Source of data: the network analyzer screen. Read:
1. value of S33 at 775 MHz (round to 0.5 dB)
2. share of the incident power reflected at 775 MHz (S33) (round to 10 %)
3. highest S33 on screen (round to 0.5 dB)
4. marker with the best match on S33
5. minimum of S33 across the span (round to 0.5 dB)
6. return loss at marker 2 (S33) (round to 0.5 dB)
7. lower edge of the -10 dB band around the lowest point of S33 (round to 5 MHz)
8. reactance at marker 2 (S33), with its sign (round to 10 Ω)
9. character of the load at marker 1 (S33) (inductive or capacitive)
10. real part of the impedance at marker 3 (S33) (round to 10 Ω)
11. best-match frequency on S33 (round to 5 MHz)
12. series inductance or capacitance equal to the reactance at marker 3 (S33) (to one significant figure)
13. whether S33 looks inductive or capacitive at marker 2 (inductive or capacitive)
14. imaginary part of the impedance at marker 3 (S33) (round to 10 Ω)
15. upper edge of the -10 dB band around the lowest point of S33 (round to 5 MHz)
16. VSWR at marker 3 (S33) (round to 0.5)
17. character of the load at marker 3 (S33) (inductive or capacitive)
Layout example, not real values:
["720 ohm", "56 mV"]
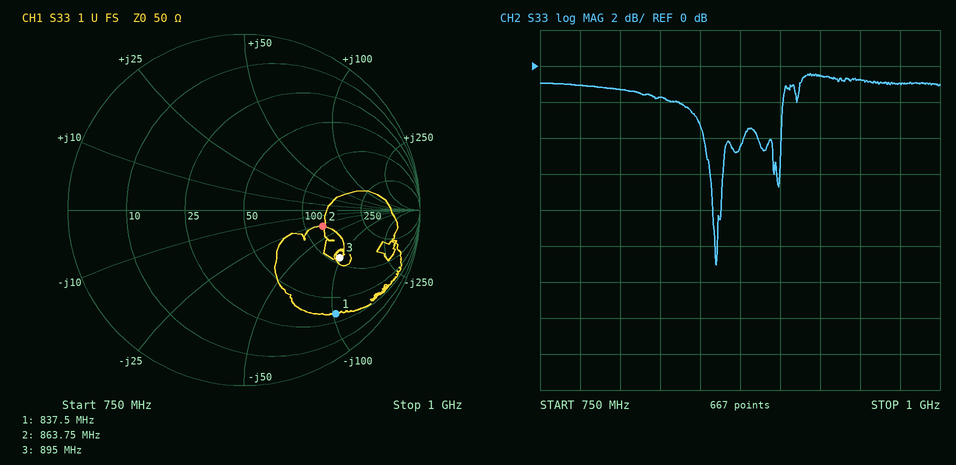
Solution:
["-1.0 dB", "80 %", "-0.5 dB", "marker 2", "-11.0 dB", "7.0 dB", "860 MHz", "-30 Ω", "capacitive", "110 Ω", "860 MHz", "2 pF", "capacitive", "-100 Ω", "860 MHz", "4.0", "capacitive"]
